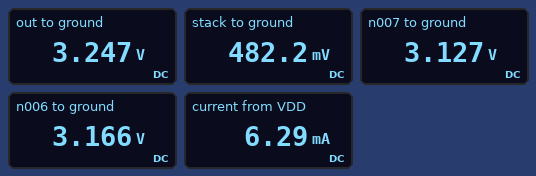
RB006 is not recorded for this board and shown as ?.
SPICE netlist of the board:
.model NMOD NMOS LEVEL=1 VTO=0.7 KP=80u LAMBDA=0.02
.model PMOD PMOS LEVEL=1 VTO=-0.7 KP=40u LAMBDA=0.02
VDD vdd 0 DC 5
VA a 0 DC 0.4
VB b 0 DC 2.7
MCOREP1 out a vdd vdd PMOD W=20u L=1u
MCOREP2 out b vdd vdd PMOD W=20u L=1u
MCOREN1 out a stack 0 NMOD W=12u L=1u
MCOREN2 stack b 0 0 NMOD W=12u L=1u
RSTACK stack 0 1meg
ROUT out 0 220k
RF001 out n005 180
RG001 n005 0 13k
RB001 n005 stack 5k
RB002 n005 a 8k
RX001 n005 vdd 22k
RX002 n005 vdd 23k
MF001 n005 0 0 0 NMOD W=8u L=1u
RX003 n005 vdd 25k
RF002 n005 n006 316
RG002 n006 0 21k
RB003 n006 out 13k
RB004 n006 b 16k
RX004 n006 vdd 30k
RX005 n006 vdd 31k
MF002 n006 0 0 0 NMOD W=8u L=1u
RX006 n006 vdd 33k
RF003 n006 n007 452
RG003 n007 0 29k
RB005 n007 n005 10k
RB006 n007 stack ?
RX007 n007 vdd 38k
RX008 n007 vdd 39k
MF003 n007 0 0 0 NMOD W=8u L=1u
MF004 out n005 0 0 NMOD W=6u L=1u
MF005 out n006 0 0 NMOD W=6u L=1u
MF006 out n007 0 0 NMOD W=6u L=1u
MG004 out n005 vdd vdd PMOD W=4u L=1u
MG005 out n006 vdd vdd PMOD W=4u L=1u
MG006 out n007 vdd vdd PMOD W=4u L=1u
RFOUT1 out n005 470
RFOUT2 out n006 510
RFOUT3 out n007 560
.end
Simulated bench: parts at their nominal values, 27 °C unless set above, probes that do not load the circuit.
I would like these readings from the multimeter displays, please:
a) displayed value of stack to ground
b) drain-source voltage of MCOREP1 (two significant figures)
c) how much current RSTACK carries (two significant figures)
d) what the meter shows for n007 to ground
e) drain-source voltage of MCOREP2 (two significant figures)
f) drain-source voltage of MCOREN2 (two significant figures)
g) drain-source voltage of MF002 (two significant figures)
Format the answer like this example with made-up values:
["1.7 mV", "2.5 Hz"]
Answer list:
["482.2 mV", "-1.8 V", "480 nA", "3.127 V", "-1.8 V", "480 mV", "3.2 V"]
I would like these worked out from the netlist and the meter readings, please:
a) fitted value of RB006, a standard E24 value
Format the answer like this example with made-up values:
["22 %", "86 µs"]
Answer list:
["9.1 kΩ"]
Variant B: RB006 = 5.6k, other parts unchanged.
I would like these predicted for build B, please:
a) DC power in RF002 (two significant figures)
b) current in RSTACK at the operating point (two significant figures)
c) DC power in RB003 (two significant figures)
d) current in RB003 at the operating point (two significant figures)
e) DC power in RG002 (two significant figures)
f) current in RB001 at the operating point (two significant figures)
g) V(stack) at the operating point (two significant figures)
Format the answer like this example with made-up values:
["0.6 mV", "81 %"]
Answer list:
["480 nW", "580 nA", "690 nW", "7.3 µA", "470 µW", "510 µA", "580 mV"]
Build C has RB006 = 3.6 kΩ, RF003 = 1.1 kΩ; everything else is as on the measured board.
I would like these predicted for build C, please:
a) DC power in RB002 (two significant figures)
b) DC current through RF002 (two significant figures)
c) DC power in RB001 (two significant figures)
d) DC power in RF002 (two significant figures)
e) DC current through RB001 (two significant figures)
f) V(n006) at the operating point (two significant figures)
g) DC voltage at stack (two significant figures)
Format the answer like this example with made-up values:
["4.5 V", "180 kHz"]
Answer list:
["930 µW", "38 µA", "1.2 mW", "460 nW", "490 µA", "3.1 V", "700 mV"]
